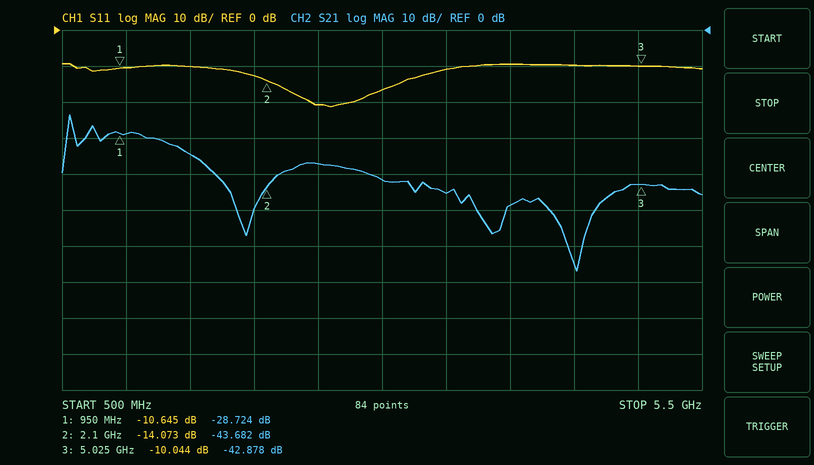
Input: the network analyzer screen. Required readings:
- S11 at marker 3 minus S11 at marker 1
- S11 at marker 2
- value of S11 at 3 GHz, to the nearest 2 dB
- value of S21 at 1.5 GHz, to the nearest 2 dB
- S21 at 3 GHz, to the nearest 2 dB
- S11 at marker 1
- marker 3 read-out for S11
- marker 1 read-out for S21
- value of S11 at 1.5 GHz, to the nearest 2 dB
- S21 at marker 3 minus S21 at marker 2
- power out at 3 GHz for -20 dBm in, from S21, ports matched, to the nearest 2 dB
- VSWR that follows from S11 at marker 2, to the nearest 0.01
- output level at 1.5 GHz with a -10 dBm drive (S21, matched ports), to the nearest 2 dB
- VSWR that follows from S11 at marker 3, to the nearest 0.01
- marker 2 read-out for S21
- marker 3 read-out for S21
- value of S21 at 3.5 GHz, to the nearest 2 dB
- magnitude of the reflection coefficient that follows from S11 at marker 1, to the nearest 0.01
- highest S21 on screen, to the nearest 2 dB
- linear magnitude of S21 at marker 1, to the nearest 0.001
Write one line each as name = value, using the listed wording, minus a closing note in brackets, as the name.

S11 at marker 3 minus S11 at marker 1 = 0.601 dB
S11 at marker 2 = -14.073 dB
value of S11 at 3 GHz, to the nearest 2 dB = -16 dB
value of S21 at 1.5 GHz, to the nearest 2 dB = -34 dB
S21 at 3 GHz, to the nearest 2 dB = -42 dB
S11 at marker 1 = -10.645 dB
marker 3 read-out for S11 = -10.044 dB
marker 1 read-out for S21 = -28.724 dB
value of S11 at 1.5 GHz, to the nearest 2 dB = -10 dB
S21 at marker 3 minus S21 at marker 2 = 0.804 dB
power out at 3 GHz for -20 dBm in, from S21, ports matched, to the nearest 2 dB = -62 dBm
VSWR that follows from S11 at marker 2, to the nearest 0.01 = 1.49
output level at 1.5 GHz with a -10 dBm drive (S21, matched ports), to the nearest 2 dB = -44 dBm
VSWR that follows from S11 at marker 3, to the nearest 0.01 = 1.92
marker 2 read-out for S21 = -43.682 dB
marker 3 read-out for S21 = -42.878 dB
value of S21 at 3.5 GHz, to the nearest 2 dB = -46 dB
magnitude of the reflection coefficient that follows from S11 at marker 1, to the nearest 0.01 = 0.29
highest S21 on screen, to the nearest 2 dB = -24 dB
linear magnitude of S21 at marker 1, to the nearest 0.001 = 0.037
